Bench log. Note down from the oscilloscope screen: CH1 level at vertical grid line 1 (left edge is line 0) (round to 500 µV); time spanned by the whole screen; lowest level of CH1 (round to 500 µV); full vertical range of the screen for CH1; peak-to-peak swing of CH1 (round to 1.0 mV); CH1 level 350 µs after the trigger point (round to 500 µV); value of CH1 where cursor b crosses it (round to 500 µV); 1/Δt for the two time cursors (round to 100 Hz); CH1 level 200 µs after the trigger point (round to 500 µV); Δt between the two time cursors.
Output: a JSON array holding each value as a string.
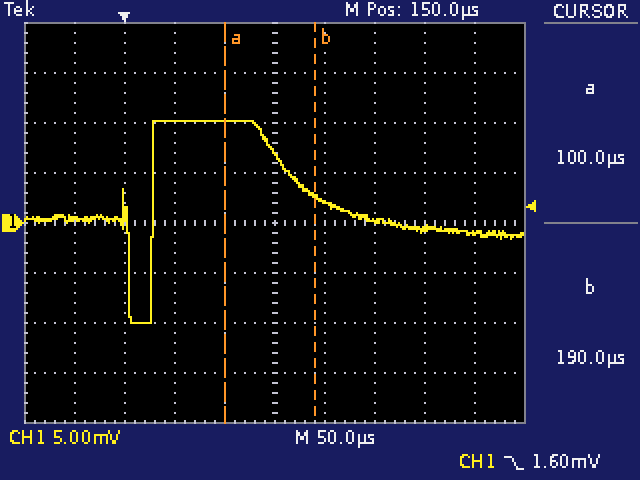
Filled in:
["500 µV", "500 µs", "-10.0 mV", "40 mV", "20.0 mV", "-1.0 mV", "2.5 mV", "11.1 kHz", "2.0 mV", "90 µs"]
